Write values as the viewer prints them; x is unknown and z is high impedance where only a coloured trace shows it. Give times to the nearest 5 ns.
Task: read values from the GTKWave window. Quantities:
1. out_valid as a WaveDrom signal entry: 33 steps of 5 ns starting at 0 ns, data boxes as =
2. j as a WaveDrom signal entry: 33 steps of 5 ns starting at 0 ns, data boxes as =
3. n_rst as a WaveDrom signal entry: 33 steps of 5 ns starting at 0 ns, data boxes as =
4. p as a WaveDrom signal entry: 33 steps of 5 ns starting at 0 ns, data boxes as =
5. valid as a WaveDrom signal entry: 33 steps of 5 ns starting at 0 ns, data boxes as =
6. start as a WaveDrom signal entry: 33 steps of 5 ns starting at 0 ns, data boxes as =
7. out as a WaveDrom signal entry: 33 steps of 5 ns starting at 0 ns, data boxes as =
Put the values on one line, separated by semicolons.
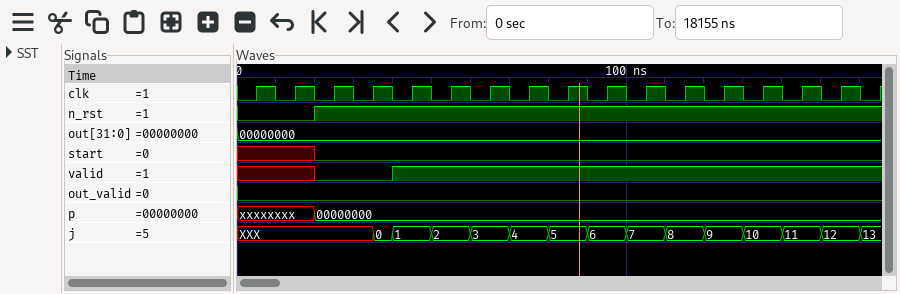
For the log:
{name: 'out_valid', wave: '0................................'}; {name: 'j', wave: 'x......==.=.=.=.=.=.=.=.=.=.=.=.=', data: '0 1 2 3 4 5 6 7 8 9 10 11 12 13'}; {name: 'n_rst', wave: '0...1............................'}; {name: 'p', wave: 'x...=............................', data: '00000000'}; {name: 'valid', wave: 'x...0...1........................'}; {name: 'start', wave: 'x...0............................'}; {name: 'out', wave: '=................................', data: '00000000'}
